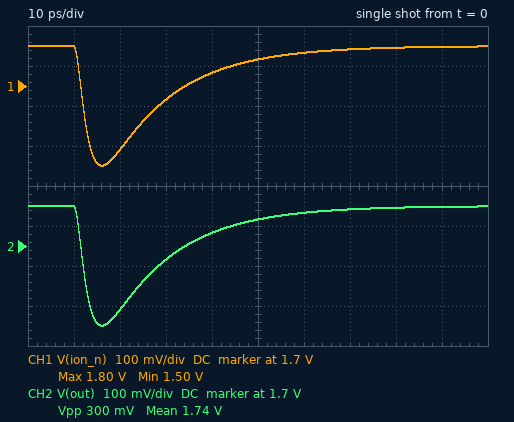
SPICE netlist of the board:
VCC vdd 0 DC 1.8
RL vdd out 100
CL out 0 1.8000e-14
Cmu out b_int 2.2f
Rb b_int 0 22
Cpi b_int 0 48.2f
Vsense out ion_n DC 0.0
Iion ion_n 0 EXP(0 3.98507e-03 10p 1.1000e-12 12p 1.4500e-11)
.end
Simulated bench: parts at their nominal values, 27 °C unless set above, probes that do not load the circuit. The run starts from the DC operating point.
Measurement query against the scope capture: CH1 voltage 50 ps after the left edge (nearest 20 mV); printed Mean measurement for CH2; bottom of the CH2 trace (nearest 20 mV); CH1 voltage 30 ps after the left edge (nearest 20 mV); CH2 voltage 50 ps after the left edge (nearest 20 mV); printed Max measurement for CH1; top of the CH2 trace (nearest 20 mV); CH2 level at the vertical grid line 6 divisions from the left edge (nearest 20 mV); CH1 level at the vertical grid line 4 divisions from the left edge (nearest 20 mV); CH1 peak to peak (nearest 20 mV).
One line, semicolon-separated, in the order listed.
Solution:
1.76 V; 1.74 V; 1.50 V; 1.66 V; 1.76 V; 1.80 V; 1.80 V; 1.78 V; 1.74 V; 300 mV
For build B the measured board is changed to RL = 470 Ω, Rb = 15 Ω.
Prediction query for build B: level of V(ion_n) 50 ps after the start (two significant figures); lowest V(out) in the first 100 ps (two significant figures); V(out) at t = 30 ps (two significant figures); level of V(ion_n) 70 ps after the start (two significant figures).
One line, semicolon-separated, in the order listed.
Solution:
1.5 V; 910 mV; 1.0 V; 1.7 V
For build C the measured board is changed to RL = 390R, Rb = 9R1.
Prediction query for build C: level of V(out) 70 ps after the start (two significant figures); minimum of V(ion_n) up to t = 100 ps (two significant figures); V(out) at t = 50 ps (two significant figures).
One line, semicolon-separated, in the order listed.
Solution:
1.7 V; 1.0 V; 1.6 V
